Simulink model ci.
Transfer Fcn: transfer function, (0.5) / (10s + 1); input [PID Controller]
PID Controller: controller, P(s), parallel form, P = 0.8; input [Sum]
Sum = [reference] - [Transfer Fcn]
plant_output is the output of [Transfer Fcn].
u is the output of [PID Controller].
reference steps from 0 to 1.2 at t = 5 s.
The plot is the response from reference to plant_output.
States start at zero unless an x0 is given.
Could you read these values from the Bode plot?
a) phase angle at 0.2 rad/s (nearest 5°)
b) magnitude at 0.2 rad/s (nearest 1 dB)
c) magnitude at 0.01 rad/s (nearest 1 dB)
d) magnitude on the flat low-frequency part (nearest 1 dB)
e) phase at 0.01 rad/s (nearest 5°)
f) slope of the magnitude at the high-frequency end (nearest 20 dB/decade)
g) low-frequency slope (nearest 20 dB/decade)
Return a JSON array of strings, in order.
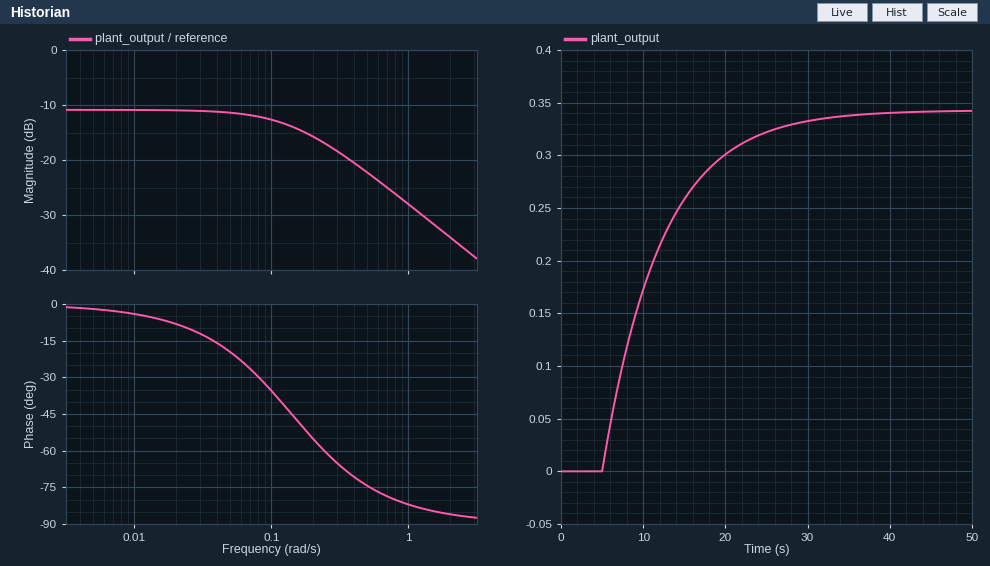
["-55°", "-16 dB", "-11 dB", "-11 dB", "-5°", "-20 dB/decade", "0 dB/decade"]
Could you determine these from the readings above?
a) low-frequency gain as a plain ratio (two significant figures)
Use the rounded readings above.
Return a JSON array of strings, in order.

["0.28"]
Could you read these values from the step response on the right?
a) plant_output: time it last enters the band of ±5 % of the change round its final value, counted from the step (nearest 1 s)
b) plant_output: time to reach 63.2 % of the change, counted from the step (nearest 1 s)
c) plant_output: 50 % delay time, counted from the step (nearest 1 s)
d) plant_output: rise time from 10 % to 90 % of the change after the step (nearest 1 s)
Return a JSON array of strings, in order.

["21 s", "7 s", "5 s", "16 s"]
